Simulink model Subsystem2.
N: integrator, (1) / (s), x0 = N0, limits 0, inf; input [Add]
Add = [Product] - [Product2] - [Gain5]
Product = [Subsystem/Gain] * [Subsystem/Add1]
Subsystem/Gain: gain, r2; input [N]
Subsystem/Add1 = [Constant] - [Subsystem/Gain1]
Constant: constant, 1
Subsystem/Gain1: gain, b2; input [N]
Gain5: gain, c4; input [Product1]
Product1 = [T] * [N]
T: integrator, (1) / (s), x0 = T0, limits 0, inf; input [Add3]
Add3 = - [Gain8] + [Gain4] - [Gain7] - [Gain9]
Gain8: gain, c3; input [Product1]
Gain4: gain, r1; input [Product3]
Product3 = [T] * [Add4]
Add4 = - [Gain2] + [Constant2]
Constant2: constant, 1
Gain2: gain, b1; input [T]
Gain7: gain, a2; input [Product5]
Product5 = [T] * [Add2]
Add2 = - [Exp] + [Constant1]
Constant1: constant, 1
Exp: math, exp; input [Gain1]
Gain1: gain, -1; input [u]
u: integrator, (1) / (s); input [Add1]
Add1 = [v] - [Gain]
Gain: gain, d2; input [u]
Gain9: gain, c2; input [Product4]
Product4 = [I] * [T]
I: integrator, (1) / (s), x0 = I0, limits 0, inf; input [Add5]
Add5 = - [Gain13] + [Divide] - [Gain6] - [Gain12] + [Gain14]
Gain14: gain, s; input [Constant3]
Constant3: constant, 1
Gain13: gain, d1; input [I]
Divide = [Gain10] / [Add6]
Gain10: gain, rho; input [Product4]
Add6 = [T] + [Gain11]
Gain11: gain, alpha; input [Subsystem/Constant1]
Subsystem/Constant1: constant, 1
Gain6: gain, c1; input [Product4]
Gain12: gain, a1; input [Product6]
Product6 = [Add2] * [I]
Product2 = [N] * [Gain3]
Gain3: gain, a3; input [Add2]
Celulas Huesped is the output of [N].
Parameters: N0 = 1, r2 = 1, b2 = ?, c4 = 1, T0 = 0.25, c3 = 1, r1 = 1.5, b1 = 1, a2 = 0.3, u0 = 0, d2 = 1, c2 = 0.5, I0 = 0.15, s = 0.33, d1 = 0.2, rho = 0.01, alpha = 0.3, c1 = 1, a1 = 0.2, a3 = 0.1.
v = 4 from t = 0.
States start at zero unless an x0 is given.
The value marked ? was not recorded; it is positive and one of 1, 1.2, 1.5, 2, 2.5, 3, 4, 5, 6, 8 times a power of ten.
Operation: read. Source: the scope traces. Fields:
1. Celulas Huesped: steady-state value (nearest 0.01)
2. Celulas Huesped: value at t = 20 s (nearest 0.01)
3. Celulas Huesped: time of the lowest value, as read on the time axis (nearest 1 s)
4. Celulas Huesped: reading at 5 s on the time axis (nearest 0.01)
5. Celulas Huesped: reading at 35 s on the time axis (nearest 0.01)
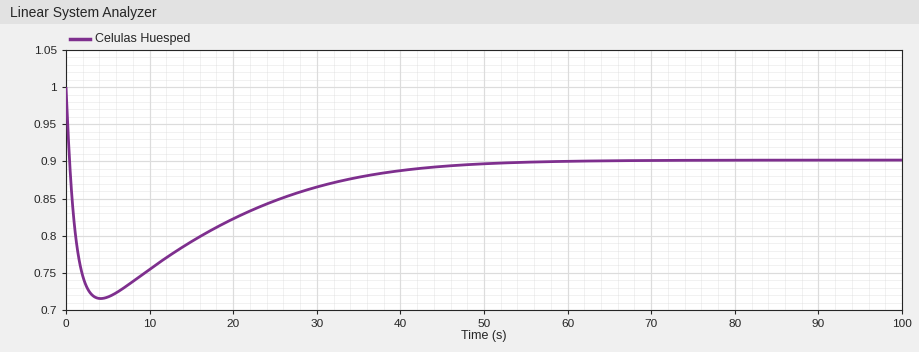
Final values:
0.90
0.82
4 s
0.72
0.88
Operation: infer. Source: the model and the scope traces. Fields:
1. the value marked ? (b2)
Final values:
1
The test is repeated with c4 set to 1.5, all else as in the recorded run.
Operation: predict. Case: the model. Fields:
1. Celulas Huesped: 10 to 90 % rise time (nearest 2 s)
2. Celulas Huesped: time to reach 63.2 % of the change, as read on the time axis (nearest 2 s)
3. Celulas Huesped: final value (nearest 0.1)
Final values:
34 s
20 s
0.0
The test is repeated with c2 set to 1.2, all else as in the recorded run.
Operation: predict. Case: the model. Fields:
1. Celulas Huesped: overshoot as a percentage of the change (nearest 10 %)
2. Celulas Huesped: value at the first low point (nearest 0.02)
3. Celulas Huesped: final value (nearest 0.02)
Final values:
130 %
0.78
0.90
